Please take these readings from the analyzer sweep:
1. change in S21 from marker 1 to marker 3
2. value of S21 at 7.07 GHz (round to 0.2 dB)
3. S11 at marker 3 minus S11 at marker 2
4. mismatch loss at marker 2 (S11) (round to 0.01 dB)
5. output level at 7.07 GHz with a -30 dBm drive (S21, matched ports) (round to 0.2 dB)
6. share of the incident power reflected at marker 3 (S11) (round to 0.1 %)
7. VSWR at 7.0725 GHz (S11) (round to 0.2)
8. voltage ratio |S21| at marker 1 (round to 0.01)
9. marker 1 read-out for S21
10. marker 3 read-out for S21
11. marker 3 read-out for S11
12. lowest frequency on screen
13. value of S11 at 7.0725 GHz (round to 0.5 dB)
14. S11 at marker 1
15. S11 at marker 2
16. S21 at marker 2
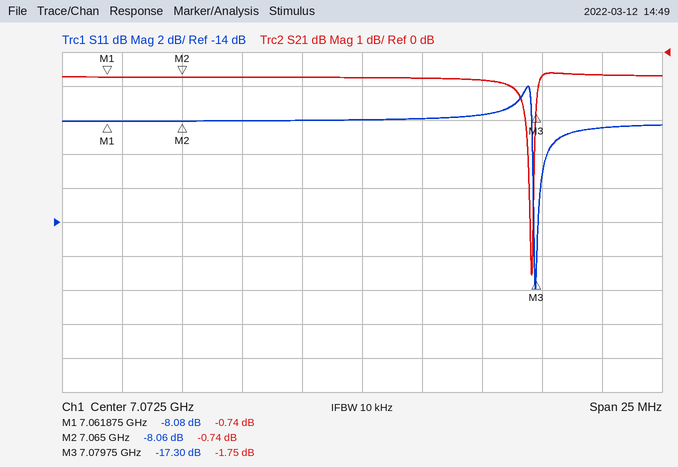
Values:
-1.01 dB
-0.8 dB
-9.24 dB
0.74 dB
-30.8 dBm
1.9 %
2.4
0.92
-0.74 dB
-1.75 dB
-17.30 dB
7.06 GHz
-8.0 dB
-8.08 dB
-8.06 dB
-0.74 dB
